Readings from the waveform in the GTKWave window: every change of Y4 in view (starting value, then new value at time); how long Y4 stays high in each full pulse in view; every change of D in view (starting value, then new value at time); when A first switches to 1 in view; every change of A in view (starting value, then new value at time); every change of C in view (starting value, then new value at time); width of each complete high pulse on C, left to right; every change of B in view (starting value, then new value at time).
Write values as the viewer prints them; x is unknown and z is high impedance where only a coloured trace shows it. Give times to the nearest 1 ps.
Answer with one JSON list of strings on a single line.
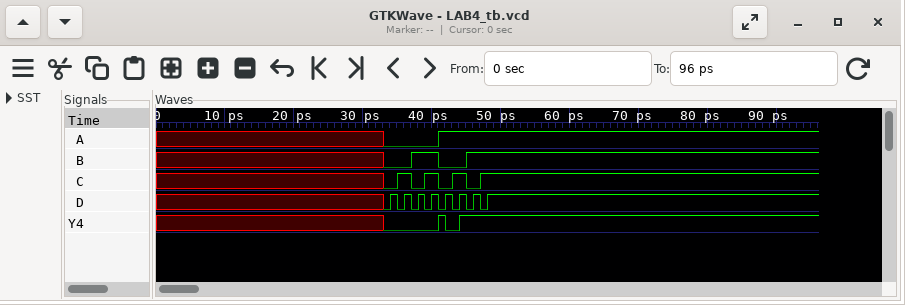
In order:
["x, 0 at 33 ps, 1 at 41 ps, 0 at 42 ps, 1 at 44 ps", "1 ps", "x, 0 at 33 ps, 1 at 34 ps, 0 at 35 ps, 1 at 36 ps, 0 at 37 ps, 1 at 38 ps, 0 at 39 ps, 1 at 40 ps, 0 at 41 ps, 1 at 42 ps, 0 at 43 ps, 1 at 44 ps, 0 at 45 ps, 1 at 46 ps, 0 at 47 ps, 1 at 48 ps", "41 ps", "x, 0 at 33 ps, 1 at 41 ps", "x, 0 at 33 ps, 1 at 35 ps, 0 at 37 ps, 1 at 39 ps, 0 at 41 ps, 1 at 43 ps, 0 at 45 ps, 1 at 47 ps", "2 ps, 2 ps, 2 ps", "x, 0 at 33 ps, 1 at 37 ps, 0 at 41 ps, 1 at 45 ps"]
